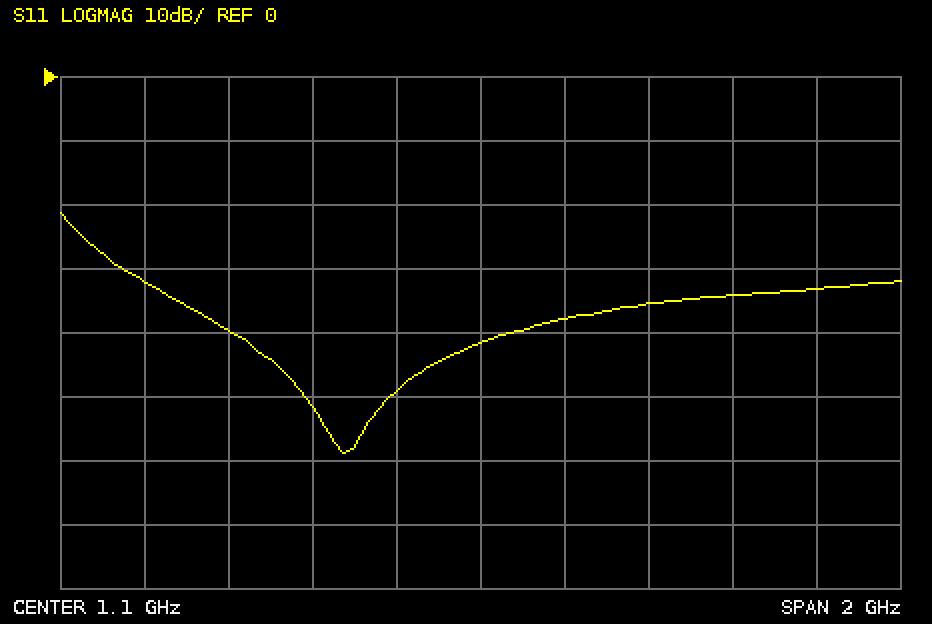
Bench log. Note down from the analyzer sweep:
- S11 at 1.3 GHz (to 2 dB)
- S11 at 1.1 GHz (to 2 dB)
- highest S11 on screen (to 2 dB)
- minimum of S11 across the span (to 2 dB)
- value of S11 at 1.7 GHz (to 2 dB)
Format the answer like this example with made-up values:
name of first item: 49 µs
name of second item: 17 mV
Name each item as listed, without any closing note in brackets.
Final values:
S11 at 1.3 GHz: -38 dB
S11 at 1.1 GHz: -42 dB
highest S11 on screen: -22 dB
minimum of S11 across the span: -58 dB
value of S11 at 1.7 GHz: -34 dB
